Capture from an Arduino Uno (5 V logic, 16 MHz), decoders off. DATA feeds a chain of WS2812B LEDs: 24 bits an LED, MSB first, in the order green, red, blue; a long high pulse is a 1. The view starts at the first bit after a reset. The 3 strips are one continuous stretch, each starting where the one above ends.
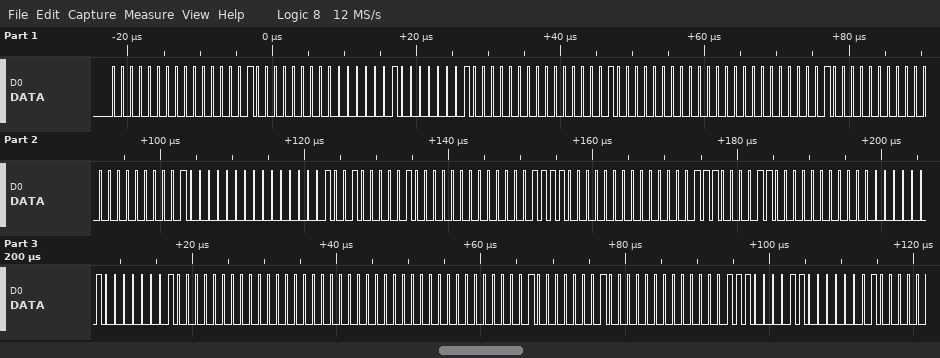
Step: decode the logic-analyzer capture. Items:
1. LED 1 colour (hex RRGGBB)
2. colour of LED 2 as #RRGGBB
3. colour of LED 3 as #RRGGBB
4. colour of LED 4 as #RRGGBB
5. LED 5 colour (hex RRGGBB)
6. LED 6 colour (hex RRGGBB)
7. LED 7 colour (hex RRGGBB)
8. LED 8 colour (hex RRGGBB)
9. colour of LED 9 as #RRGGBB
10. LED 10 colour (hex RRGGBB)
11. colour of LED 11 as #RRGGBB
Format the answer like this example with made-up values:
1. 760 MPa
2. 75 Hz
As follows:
1. #010000
2. #010100
3. #000100
4. #000100
5. #000809
6. #00041E
7. #07000C
8. #010001
9. #000000
10. #010001
11. #07000C
